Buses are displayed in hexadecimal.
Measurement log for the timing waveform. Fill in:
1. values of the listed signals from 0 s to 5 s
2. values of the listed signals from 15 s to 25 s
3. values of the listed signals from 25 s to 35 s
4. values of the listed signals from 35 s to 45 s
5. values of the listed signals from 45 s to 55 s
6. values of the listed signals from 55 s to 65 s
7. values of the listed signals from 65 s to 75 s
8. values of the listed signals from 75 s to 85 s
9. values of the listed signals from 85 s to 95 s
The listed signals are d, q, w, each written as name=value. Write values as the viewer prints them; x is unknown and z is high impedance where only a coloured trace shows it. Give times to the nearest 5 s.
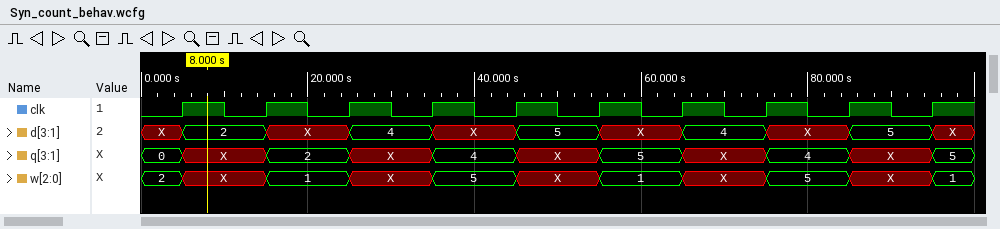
d=X, q=0, w=2
d=X, q=2, w=1
d=4, q=X, w=X
d=X, q=4, w=5
d=5, q=X, w=X
d=X, q=5, w=1
d=4, q=X, w=X
d=X, q=4, w=5
d=5, q=X, w=X
